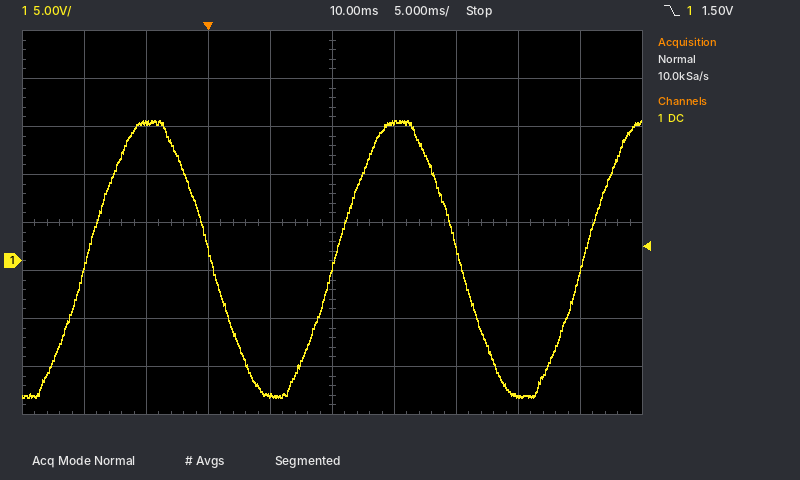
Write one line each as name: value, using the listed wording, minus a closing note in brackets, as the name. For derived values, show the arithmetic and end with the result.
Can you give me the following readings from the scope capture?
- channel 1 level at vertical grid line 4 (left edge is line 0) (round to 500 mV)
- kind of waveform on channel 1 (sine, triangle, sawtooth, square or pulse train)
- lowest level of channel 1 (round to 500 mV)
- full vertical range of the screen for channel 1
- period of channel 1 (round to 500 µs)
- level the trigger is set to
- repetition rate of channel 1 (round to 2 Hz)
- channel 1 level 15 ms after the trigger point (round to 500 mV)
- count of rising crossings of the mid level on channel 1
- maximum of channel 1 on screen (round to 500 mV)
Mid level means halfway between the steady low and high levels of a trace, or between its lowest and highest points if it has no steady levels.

channel 1 level at vertical grid line 4 (left edge is line 0): -14.0 V
kind of waveform on channel 1: sine
lowest level of channel 1: -14.0 V
full vertical range of the screen for channel 1: 40 V
period of channel 1: 20.0 ms
level the trigger is set to: 1.50 V
repetition rate of channel 1: 1 / 20.0 ms ≈ 50 Hz
channel 1 level 15 ms after the trigger point: 14.5 V
count of rising crossings of the mid level on channel 1: 3
maximum of channel 1 on screen: 14.5 V
